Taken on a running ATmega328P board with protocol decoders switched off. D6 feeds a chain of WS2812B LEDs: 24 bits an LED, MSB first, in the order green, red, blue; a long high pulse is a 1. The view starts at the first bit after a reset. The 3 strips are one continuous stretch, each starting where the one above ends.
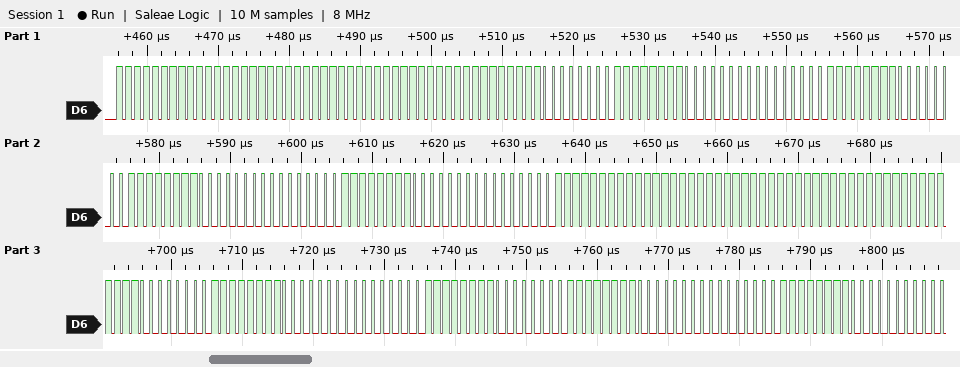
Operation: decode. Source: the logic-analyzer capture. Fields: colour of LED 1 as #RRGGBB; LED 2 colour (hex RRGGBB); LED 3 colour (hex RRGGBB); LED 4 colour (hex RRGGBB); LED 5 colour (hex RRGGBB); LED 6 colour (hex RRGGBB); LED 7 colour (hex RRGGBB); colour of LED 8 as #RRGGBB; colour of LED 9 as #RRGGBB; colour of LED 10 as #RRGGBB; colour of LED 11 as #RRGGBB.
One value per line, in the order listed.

#FFFFFF
#FFFFFF
#FF0000
#FF0000
#00FF00
#00FF00
#FFFFFF
#FFFFFF
#FF0000
#FF0000
#00FF00
